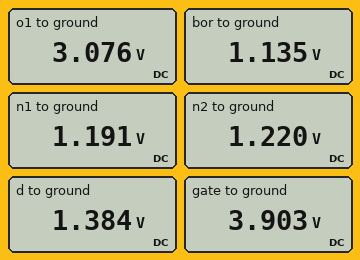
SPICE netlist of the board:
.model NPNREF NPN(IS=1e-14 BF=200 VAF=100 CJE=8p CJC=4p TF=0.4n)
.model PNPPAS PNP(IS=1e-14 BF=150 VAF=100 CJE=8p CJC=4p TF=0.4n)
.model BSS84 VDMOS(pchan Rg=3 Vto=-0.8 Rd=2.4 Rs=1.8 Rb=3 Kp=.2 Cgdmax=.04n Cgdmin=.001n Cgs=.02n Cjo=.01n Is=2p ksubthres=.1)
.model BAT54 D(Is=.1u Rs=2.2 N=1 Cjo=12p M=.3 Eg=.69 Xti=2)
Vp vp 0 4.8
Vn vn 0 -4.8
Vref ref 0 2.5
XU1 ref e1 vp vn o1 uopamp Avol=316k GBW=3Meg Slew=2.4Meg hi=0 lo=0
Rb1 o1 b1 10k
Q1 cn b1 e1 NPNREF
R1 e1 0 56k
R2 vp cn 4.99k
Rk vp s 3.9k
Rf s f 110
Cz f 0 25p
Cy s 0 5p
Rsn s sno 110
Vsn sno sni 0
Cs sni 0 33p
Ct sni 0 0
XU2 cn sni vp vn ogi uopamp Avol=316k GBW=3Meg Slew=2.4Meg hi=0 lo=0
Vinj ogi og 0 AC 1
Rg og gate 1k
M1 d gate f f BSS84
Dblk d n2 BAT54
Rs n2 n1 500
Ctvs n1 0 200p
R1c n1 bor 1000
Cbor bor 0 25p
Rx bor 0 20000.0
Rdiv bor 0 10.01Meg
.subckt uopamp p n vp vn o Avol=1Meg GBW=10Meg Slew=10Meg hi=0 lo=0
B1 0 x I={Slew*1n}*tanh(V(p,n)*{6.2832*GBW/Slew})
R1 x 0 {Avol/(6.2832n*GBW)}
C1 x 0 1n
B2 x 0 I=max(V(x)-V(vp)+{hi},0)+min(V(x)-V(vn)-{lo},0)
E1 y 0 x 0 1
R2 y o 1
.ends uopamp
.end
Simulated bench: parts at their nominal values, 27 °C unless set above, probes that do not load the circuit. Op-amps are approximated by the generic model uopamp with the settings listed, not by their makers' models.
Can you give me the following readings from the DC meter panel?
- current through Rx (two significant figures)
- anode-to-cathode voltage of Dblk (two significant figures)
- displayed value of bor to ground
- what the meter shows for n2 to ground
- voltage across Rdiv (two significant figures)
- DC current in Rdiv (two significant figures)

57 µA
160 mV
1.135 V
1.220 V
1.1 V
110 nA
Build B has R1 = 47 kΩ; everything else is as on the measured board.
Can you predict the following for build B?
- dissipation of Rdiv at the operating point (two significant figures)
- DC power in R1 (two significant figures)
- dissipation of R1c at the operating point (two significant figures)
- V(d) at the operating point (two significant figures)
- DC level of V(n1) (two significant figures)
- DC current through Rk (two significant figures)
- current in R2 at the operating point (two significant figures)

180 nW
130 µW
4.6 µW
1.6 V
1.4 V
68 µA
53 µA
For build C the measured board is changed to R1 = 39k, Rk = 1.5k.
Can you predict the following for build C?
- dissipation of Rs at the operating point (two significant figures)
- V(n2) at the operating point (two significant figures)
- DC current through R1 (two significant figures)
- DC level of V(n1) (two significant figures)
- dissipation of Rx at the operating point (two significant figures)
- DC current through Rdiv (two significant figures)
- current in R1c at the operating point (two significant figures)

20 µW
4.3 V
64 µA
4.2 V
790 µW
400 nA
200 µA
